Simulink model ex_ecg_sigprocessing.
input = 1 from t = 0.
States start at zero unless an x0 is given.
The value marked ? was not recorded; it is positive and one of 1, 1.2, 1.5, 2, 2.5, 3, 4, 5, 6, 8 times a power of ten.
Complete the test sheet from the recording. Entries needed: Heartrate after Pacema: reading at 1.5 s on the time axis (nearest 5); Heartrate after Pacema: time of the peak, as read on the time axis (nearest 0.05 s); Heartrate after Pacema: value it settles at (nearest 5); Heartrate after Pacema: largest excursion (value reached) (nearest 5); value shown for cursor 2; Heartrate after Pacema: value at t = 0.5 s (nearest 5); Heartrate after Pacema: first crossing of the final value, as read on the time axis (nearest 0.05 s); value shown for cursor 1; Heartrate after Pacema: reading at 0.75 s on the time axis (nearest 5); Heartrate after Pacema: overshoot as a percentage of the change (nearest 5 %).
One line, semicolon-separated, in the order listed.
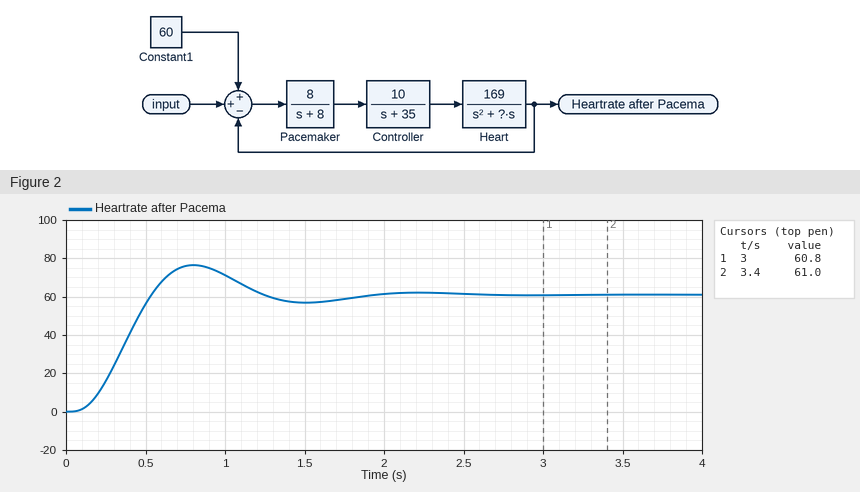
55; 0.80 s; 60; 75; 61.0; 55; 0.55 s; 60.8; 75; 25 %
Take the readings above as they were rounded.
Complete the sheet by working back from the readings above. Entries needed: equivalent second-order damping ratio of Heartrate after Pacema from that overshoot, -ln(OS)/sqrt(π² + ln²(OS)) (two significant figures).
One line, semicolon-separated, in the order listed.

0.40
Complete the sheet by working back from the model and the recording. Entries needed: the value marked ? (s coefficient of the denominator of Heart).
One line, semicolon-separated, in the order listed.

12
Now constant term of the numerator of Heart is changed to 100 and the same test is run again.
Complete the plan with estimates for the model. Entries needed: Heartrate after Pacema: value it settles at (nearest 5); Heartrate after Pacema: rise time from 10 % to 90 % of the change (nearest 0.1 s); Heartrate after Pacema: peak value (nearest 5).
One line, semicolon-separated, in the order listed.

60; 0.5 s; 65
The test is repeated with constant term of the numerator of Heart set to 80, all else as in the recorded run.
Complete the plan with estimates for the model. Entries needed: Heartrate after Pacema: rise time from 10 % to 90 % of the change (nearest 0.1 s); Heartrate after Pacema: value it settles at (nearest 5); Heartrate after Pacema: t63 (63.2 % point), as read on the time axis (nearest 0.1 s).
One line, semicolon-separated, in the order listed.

0.7 s; 60; 0.6 s
